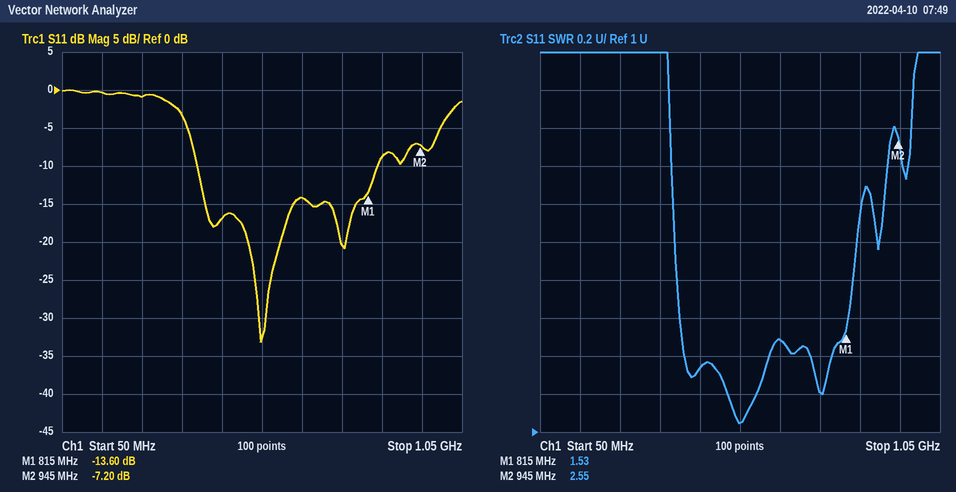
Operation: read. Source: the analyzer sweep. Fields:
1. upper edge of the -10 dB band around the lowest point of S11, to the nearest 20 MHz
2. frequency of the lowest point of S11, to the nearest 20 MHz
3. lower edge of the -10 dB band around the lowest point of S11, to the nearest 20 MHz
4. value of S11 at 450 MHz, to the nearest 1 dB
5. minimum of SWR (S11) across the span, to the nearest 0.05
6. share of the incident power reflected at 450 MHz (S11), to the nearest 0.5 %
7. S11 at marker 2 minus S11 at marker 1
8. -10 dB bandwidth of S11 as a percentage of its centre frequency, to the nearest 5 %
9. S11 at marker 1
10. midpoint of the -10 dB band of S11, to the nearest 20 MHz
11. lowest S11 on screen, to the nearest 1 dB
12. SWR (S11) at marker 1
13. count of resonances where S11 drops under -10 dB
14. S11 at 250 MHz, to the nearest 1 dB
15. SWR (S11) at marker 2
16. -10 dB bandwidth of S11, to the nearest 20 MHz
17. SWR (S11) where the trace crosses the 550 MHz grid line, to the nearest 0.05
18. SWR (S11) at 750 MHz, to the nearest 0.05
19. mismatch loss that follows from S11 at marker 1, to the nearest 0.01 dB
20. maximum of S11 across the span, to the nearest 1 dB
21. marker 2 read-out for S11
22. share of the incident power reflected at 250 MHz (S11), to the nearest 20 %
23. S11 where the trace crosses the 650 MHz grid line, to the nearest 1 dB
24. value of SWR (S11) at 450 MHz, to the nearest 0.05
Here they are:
840 MHz
540 MHz
380 MHz
-17 dB
1.05
2.0 %
6.40 dB
75 %
-13.60 dB
620 MHz
-33 dB
1.53
2
-1 dB
2.55
460 MHz
1.05
1.20
0.19 dB
0 dB
-7.20 dB
80 %
-14 dB
1.35
